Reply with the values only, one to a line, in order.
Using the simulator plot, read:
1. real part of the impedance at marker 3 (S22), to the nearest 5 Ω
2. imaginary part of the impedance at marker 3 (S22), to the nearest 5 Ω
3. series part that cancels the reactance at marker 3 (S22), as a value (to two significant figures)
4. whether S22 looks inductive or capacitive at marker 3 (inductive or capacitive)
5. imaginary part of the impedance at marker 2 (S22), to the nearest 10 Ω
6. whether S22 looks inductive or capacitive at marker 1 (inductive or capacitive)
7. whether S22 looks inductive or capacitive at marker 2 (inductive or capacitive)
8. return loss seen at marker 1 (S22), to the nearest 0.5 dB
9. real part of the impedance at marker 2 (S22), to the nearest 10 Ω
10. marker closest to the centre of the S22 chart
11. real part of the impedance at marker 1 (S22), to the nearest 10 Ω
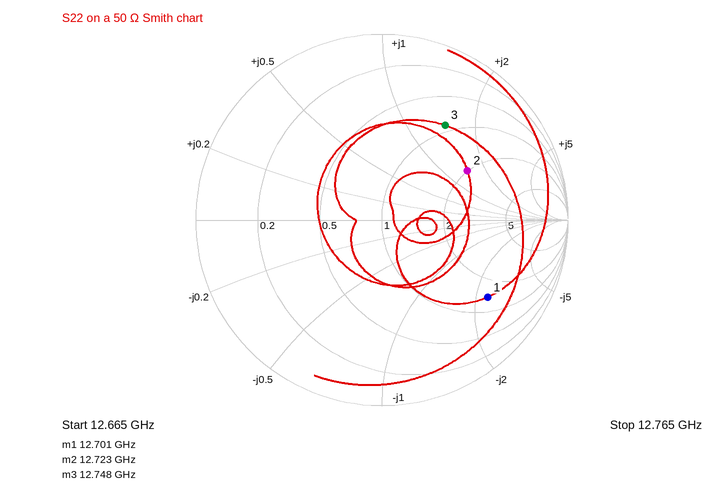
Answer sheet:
45 Ω
+75 Ω
170 fF
inductive
+70 Ω
capacitive
inductive
3.0 dB
100 Ω
marker 2
70 Ω
